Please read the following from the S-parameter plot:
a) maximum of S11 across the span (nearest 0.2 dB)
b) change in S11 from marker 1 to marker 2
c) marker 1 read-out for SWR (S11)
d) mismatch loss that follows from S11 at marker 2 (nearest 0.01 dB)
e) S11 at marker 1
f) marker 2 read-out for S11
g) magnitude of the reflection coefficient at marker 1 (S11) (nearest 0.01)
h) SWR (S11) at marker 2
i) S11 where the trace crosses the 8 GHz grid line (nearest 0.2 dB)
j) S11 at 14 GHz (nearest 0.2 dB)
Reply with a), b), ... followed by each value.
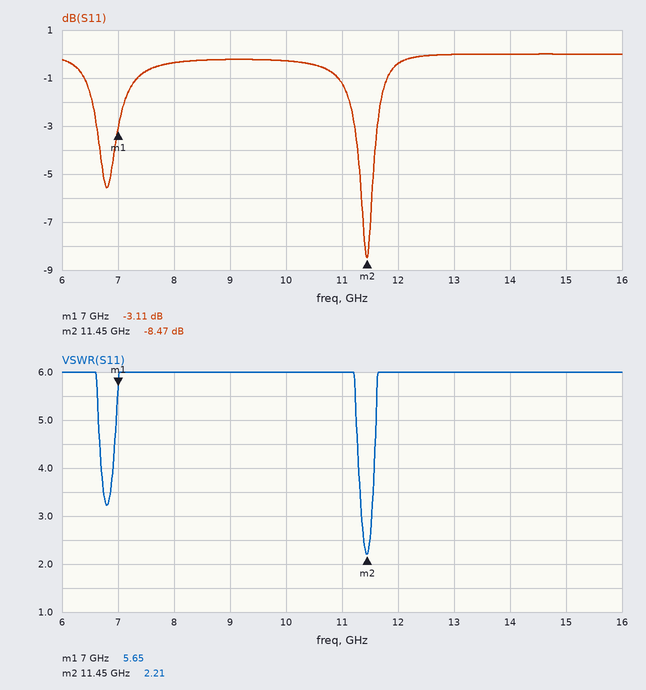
a) 0.0 dB
b) -5.36 dB
c) 5.65
d) 0.67 dB
e) -3.11 dB
f) -8.47 dB
g) 0.70
h) 2.21
i) -0.4 dB
j) 0.0 dB
